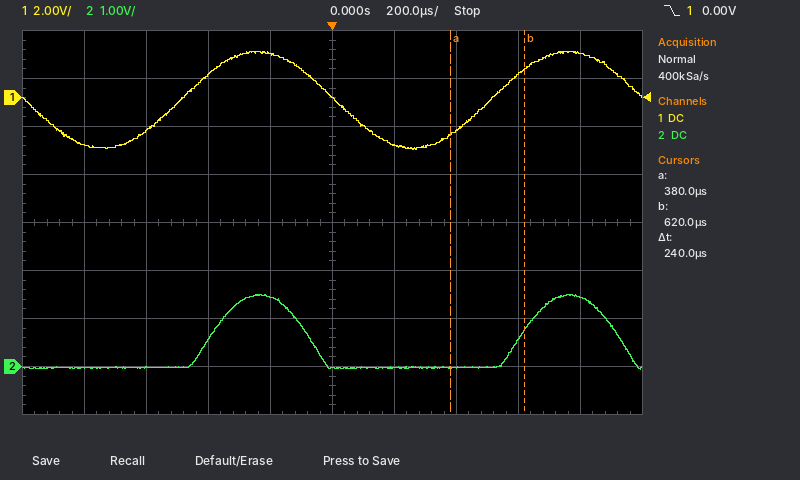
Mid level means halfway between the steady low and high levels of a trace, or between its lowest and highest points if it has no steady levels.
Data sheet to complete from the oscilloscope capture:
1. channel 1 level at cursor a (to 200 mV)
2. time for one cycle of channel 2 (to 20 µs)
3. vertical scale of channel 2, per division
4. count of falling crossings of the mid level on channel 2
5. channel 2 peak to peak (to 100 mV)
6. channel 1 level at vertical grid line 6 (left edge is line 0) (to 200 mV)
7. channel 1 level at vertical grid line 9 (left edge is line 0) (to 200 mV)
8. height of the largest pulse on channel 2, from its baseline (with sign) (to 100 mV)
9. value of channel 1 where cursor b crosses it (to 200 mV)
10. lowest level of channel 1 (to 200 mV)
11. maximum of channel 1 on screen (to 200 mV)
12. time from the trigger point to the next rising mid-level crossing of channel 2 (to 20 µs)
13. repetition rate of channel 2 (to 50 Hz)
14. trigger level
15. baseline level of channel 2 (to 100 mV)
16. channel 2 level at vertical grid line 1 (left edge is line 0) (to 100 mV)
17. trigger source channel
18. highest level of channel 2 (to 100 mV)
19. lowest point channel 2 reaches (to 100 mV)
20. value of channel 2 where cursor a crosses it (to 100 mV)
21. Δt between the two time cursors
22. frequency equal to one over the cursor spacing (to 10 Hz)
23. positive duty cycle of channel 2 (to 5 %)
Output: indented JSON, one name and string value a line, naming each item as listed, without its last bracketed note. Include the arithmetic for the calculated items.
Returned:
{
  "channel 1 level at cursor a": "-1.6 V",
  "time for one cycle of channel 2": "1.00 ms",
  "vertical scale of channel 2, per division": "1 V",
  "count of falling crossings of the mid level on channel 2": "2",
  "channel 2 peak to peak": "1.5 V − (-100 mV) = 1.6 V",
  "channel 1 level at vertical grid line 6 (left edge is line 0)": "-2.0 V",
  "channel 1 level at vertical grid line 9 (left edge is line 0)": "1.8 V",
  "height of the largest pulse on channel 2, from its baseline (with sign)": "1.5 V − (0.0 V) = +1.5 V",
  "value of channel 1 where cursor b crosses it": "1.2 V",
  "lowest level of channel 1": "-2.2 V",
  "maximum of channel 1 on screen": "2.0 V",
  "time from the trigger point to the next rising mid-level crossing of channel 2": "620 µs",
  "repetition rate of channel 2": "1 / 1.00 ms ≈ 1.00 kHz",
  "trigger level": "0.00 V",
  "baseline level of channel 2": "0.0 V",
  "channel 2 level at vertical grid line 1 (left edge is line 0)": "0.0 V",
  "trigger source channel": "channel 1",
  "highest level of channel 2": "1.5 V",
  "lowest point channel 2 reaches": "-100 mV",
  "value of channel 2 where cursor a crosses it": "0.0 V",
  "Δt between the two time cursors": "240 µs",
  "frequency equal to one over the cursor spacing": "1 / 240 µs ≈ 4.17 kHz",
  "positive duty cycle of channel 2": "30 %"
}
